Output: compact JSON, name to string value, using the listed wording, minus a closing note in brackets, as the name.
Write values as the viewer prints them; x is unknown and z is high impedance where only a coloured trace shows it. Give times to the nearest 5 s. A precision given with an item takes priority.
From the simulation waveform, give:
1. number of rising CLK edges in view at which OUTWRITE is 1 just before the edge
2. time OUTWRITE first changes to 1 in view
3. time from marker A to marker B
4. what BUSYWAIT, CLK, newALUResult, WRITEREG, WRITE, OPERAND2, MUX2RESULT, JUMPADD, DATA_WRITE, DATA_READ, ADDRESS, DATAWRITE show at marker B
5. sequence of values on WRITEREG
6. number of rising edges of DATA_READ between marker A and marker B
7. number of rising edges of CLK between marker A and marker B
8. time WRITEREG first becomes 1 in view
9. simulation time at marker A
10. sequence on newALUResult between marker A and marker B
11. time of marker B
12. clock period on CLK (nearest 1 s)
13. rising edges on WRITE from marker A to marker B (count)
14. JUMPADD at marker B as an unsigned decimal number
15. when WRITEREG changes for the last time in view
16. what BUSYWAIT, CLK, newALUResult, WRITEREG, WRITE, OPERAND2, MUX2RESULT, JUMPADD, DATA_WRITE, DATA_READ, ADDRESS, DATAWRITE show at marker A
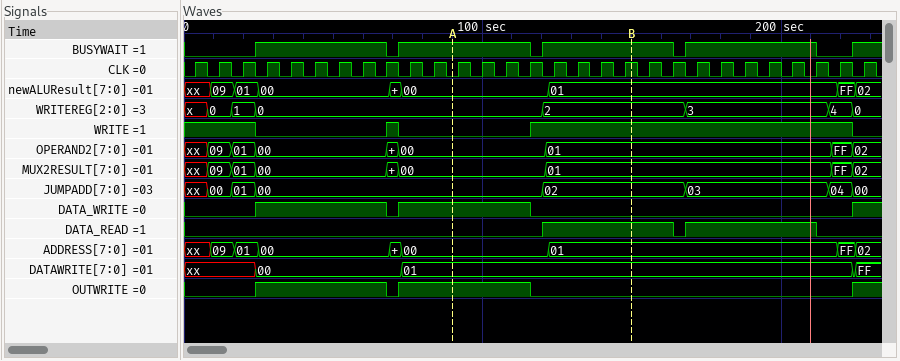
{"number of rising CLK edges in view at which OUTWRITE is 1 just before the edge": "13", "time OUTWRITE first changes to 1 in view": "25 s", "time from marker A to marker B": "60 s", "what BUSYWAIT, CLK, newALUResult, WRITEREG, WRITE, OPERAND2, MUX2RESULT, JUMPADD, DATA_WRITE, DATA_READ, ADDRESS, DATAWRITE show at marker B": "BUSYWAIT=1, CLK=1, newALUResult=01, WRITEREG=2, WRITE=1, OPERAND2=01, MUX2RESULT=01, JUMPADD=02, DATA_WRITE=0, DATA_READ=1, ADDRESS=01, DATAWRITE=01", "sequence of values on WRITEREG": "x, 0, 1, 0, 2, 3, 4, 0", "number of rising edges of DATA_READ between marker A and marker B": "1", "number of rising edges of CLK between marker A and marker B": "8", "time WRITEREG first becomes 1 in view": "15 s", "simulation time at marker A": "90 s", "sequence on newALUResult between marker A and marker B": "00, 01", "time of marker B": "150 s", "clock period on CLK": "8 s", "rising edges on WRITE from marker A to marker B": "1", "JUMPADD at marker B as an unsigned decimal number": "2", "when WRITEREG changes for the last time in view": "225 s", "what BUSYWAIT, CLK, newALUResult, WRITEREG, WRITE, OPERAND2, MUX2RESULT, JUMPADD, DATA_WRITE, DATA_READ, ADDRESS, DATAWRITE show at marker A": "BUSYWAIT=1, CLK=0, newALUResult=00, WRITEREG=0, WRITE=0, OPERAND2=00, MUX2RESULT=00, JUMPADD=00, DATA_WRITE=1, DATA_READ=0, ADDRESS=00, DATAWRITE=01"}
